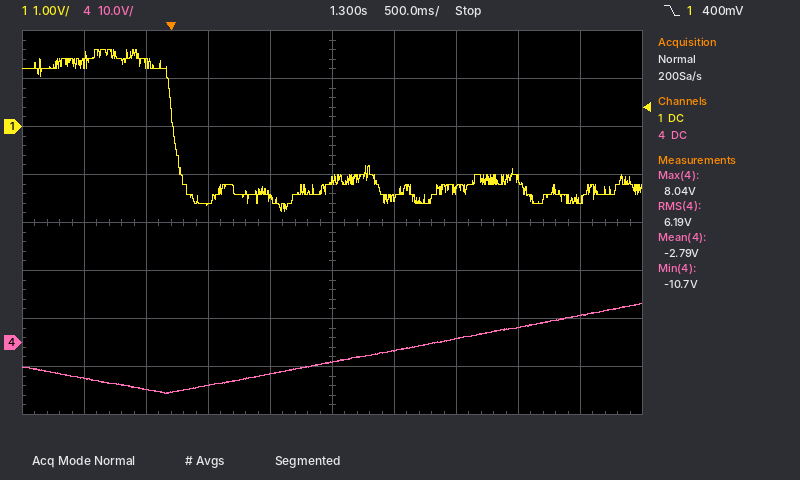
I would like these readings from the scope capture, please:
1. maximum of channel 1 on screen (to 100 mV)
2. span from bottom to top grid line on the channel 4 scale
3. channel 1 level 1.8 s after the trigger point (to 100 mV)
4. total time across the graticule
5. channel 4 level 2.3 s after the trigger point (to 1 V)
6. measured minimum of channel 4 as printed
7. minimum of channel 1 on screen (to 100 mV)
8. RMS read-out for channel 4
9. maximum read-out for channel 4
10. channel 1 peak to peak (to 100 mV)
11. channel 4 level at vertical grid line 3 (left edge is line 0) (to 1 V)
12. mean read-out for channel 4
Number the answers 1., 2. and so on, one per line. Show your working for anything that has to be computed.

1. 1.6 V
2. 80 V
3. -1.5 V
4. 5 s
5. 1 V
6. -10.7 V
7. -1.8 V
8. 6.19 V
9. 8.04 V
10. 1.6 V − (-1.8 V) = 3.4 V
11. -9 V
12. -2.79 V
